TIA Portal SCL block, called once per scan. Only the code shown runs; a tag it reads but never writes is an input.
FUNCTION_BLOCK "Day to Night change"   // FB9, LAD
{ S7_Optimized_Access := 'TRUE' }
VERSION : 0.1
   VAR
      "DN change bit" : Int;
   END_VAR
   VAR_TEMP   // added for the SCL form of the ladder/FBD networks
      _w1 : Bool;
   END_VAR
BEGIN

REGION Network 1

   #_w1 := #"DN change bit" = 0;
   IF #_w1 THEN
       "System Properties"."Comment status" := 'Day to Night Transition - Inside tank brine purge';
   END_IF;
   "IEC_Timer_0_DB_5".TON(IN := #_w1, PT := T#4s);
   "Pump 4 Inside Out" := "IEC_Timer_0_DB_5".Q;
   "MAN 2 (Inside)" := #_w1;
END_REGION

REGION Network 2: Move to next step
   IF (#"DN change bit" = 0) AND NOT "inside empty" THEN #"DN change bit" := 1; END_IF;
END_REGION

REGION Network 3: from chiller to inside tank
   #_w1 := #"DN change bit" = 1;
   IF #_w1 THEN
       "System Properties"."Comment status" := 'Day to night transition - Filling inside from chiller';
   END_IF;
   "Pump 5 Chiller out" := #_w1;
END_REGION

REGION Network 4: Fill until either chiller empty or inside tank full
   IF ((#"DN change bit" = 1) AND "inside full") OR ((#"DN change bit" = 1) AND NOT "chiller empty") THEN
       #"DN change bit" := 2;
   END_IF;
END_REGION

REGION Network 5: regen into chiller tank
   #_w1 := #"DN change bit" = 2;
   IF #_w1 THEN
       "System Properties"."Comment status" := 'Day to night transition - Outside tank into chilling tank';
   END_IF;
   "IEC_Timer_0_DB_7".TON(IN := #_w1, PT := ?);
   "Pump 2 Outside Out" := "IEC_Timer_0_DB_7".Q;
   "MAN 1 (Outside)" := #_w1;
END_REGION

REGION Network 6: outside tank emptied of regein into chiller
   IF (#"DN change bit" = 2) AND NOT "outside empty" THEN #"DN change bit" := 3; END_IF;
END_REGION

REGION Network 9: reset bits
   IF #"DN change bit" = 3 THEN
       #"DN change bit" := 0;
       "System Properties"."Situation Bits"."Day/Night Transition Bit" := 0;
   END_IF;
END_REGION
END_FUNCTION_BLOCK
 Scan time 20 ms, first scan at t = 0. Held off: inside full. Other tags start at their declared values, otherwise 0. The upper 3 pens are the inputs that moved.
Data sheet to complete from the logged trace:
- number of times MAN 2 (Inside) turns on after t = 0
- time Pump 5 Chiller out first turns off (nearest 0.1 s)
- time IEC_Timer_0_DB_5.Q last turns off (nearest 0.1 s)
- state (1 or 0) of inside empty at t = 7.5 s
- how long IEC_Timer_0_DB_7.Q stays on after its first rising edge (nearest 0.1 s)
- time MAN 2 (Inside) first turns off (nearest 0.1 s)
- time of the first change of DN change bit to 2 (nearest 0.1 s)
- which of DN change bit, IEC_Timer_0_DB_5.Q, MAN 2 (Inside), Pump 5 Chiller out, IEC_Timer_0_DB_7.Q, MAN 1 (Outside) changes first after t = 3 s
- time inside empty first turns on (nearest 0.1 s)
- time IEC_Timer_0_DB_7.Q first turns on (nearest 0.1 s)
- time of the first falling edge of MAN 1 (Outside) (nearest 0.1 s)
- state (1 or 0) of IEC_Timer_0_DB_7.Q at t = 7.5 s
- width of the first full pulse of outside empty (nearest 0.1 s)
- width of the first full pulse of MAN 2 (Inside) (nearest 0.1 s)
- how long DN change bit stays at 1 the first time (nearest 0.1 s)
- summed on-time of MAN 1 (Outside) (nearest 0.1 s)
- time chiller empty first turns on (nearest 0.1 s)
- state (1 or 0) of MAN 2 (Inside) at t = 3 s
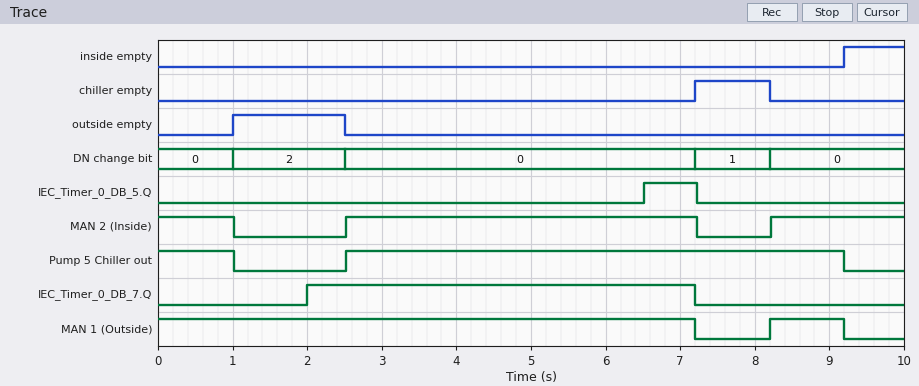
2
1.0 s
7.2 s
0
5.2 s
1.0 s
1.0 s
IEC_Timer_0_DB_5.Q
9.2 s
2.0 s
7.2 s
0
1.5 s
4.7 s
1.0 s
8.2 s
7.2 s
1
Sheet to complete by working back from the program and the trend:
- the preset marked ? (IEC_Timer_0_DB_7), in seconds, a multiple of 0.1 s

2.0 s
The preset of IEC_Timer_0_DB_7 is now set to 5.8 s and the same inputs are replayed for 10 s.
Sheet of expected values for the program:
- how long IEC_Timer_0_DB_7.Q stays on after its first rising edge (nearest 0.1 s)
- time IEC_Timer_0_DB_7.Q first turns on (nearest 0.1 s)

1.4 s
5.8 s
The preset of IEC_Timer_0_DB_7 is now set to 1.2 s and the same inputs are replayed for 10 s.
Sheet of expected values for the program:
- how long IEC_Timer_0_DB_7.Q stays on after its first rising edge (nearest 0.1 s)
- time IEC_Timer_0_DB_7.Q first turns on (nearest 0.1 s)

6.0 s
1.2 s
